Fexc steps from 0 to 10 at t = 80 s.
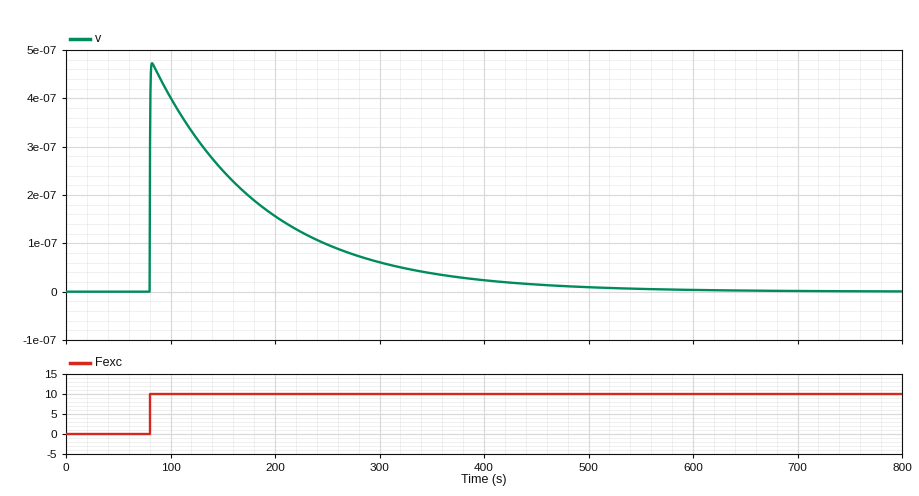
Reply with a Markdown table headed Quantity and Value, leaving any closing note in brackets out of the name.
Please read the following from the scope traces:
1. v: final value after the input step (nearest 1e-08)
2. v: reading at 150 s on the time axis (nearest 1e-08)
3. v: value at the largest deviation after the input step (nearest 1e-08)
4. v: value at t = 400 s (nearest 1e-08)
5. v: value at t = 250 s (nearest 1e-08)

| Quantity | Value |
|---|---|
| v: final value after the input step | 0.00000000 |
| v: reading at 150 s on the time axis | 0.00000025 |
| v: value at the largest deviation after the input step | 0.00000047 |
| v: value at t = 400 s | 0.00000002 |
| v: value at t = 250 s | 0.00000010 |
